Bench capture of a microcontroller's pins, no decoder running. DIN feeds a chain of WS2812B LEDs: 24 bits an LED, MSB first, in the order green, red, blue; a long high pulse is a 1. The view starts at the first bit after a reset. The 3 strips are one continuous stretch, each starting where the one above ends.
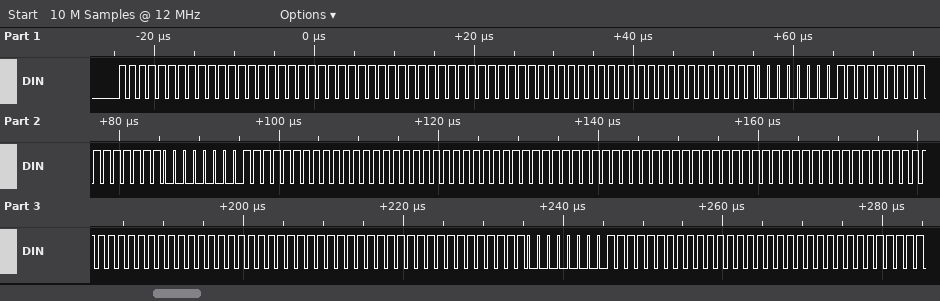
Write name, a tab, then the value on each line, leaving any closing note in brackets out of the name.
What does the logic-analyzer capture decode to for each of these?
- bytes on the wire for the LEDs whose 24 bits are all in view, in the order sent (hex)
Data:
bytes on the wire for the LEDs whose 24 bits are all in view, in the order sent	FF FF FF FF FF FF FF FF 00 FF FF 00 FF FF FF FF FF FF FF FF FF FF FF FF FF FF 00 FF FF FF
